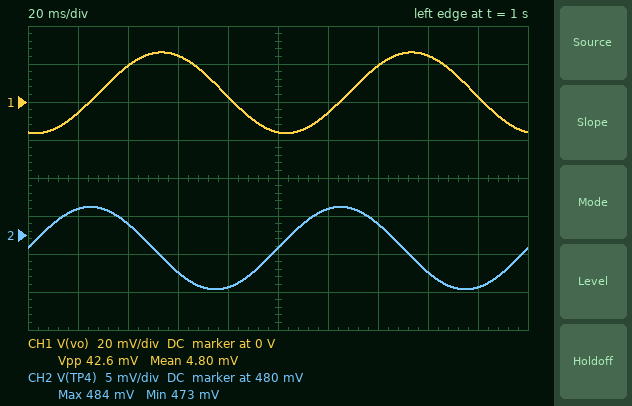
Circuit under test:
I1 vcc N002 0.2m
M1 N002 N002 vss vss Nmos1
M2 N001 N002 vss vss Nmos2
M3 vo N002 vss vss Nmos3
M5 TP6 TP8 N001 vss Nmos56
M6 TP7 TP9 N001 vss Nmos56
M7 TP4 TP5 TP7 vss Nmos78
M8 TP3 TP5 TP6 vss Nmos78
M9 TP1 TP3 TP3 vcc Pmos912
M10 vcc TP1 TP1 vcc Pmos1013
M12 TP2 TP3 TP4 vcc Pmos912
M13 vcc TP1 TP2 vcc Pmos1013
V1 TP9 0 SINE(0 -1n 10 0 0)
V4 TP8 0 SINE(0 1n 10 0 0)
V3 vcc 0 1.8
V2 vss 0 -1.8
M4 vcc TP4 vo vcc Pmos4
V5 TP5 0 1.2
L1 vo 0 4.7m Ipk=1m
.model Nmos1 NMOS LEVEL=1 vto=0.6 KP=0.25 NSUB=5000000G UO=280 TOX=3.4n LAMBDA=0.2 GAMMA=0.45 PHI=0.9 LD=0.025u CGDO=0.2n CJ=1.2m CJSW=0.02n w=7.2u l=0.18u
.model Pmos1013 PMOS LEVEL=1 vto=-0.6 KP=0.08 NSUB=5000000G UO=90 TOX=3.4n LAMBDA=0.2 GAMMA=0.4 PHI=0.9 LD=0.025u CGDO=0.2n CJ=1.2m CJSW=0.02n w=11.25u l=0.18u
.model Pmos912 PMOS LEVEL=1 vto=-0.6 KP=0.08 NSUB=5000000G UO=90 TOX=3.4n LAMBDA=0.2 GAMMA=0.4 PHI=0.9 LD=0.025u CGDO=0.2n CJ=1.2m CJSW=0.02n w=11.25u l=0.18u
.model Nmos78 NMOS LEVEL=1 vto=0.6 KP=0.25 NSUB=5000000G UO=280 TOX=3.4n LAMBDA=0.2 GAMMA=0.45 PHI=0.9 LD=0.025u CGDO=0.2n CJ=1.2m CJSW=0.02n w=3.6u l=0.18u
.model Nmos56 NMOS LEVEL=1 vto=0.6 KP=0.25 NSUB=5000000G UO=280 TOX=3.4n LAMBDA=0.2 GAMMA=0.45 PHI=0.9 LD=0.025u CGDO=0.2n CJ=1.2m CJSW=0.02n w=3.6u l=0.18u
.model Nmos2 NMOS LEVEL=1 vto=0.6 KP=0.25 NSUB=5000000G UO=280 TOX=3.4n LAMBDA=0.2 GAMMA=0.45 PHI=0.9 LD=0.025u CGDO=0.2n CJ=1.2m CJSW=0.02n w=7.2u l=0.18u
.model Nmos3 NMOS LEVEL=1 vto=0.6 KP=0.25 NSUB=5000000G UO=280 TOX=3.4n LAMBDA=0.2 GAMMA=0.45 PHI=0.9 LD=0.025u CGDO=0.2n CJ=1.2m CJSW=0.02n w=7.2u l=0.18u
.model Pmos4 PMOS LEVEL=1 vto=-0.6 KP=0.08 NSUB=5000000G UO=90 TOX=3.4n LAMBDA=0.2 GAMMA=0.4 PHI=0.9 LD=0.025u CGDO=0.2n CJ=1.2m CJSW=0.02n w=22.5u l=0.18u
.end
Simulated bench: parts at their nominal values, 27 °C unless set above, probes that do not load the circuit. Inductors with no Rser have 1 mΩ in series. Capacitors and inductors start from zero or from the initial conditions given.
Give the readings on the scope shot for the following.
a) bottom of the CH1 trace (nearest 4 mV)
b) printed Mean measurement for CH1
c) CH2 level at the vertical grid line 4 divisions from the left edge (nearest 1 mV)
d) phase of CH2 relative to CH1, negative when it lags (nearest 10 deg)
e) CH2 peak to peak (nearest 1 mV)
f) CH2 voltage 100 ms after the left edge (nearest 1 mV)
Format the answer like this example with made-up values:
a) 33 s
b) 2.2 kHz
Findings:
a) -16 mV
b) 4.80 mV
c) 473 mV
d) 100 deg
e) 11 mV
f) 478 mV
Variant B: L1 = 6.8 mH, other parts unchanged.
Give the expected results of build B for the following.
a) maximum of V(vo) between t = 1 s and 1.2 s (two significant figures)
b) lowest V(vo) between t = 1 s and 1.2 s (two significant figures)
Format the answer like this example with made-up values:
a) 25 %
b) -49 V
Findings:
a) 35 mV
b) -25 mV
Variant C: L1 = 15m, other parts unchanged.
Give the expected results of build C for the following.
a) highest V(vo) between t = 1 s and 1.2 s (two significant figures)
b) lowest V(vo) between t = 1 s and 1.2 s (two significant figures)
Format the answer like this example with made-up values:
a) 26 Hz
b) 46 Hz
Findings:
a) 62 mV
b) -53 mV
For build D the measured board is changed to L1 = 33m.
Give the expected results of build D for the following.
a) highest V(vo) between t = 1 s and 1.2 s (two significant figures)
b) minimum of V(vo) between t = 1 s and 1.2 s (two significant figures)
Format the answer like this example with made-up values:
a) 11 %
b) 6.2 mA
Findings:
a) 89 mV
b) -80 mV
